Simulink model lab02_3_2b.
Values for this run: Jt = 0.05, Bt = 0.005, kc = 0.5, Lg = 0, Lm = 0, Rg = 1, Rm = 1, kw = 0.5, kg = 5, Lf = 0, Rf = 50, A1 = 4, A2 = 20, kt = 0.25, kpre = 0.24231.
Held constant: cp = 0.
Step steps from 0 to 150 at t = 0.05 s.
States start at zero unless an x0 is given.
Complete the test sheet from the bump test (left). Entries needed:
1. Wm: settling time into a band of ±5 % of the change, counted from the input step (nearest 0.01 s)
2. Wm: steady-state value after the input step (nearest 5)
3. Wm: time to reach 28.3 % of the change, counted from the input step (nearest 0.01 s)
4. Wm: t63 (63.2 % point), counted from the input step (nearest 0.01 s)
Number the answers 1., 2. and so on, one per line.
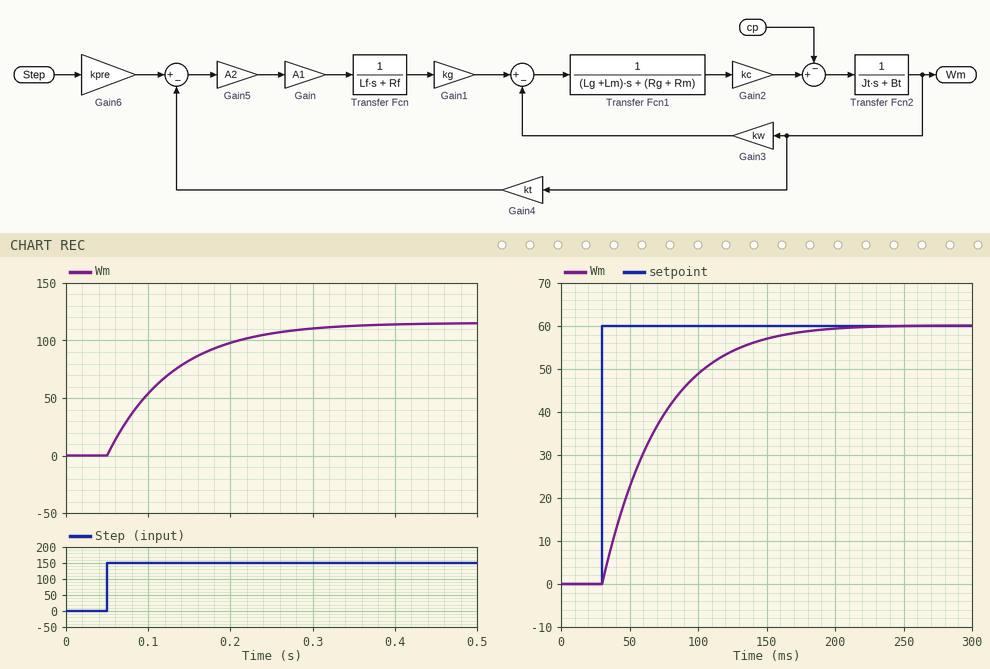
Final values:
1. 0.24 s
2. 115
3. 0.03 s
4. 0.08 s
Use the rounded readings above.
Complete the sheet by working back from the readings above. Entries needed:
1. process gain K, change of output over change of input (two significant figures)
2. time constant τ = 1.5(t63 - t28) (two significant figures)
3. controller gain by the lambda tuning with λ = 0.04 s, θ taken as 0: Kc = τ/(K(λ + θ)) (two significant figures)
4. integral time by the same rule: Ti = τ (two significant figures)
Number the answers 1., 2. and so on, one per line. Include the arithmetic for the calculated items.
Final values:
1. (115 - 0) / 150 = 0.77
2. 1.5 × (0.08 - 0.03) = 0.075 s
3. 0.075 / (0.77 × (0.04 + 0)) = 2.4
4. 0.075 s
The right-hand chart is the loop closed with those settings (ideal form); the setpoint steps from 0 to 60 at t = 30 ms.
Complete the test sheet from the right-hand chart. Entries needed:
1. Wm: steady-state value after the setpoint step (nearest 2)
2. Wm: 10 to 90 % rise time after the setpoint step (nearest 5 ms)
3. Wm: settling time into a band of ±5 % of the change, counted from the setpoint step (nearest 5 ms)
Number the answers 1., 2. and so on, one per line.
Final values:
1. 60
2. 90 ms
3. 120 ms
